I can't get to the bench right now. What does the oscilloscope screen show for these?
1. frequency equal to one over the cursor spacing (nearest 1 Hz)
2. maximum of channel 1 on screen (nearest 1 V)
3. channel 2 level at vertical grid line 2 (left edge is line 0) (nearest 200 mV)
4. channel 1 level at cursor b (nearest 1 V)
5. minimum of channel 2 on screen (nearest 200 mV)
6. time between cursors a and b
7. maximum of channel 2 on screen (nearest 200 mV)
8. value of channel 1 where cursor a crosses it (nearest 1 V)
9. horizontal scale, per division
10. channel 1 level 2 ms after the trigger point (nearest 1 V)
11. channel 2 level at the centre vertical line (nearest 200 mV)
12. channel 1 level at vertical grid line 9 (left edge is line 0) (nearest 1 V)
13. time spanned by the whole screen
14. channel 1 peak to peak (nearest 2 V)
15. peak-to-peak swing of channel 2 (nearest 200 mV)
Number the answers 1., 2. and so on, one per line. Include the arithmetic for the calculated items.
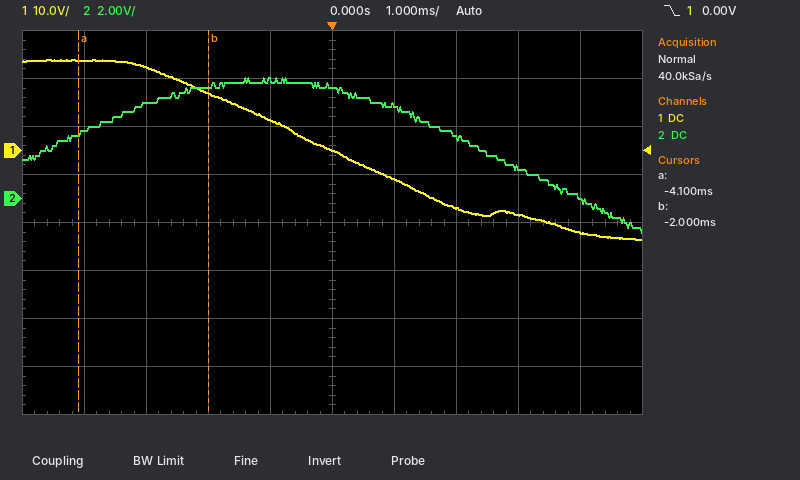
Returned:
1. 1 / 2.1 ms ≈ 476 Hz
2. 19 V
3. 4.0 V
4. 12 V
5. -1.4 V
6. -2 ms − (-4.1 ms) = 2.1 ms
7. 5.0 V
8. 19 V
9. 1 ms
10. -12 V
11. 4.6 V
12. -17 V
13. 10 ms
14. 38 V
15. 5.0 V − (-1.4 V) = 6.4 V
